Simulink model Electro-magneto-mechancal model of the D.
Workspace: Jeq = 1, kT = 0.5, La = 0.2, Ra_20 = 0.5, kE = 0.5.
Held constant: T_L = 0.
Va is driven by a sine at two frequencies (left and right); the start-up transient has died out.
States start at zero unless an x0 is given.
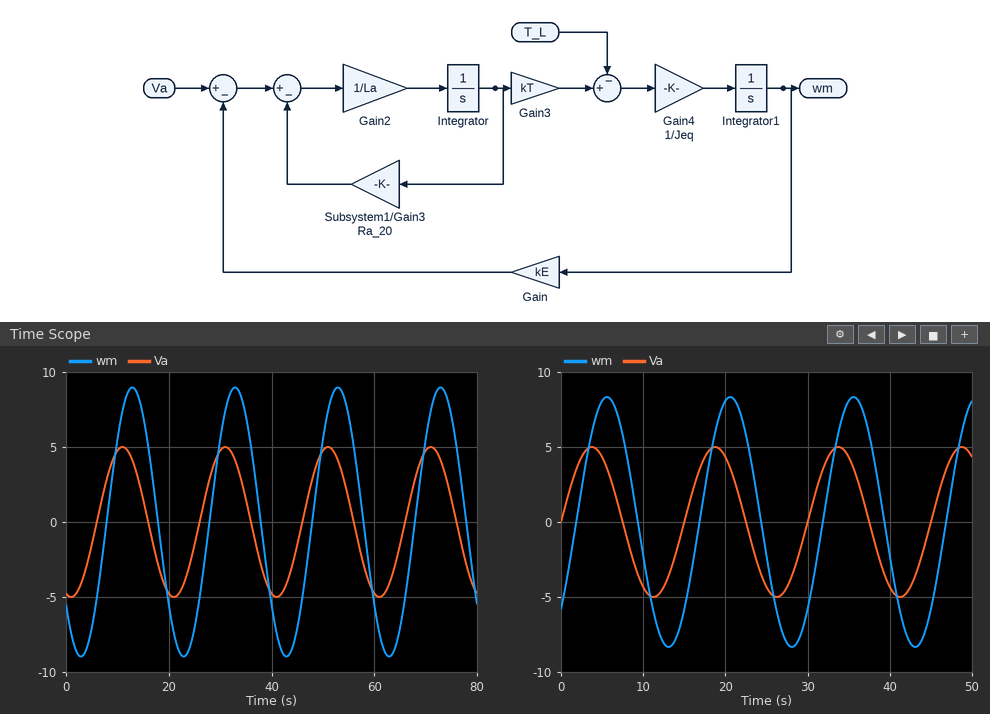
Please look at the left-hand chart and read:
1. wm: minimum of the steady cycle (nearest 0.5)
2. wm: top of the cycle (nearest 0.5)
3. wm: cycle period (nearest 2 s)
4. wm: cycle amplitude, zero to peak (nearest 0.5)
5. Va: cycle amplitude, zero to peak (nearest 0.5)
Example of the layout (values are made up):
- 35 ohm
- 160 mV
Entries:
- -9.0
- 9.0
- 20 s
- 9.0
- 5.0
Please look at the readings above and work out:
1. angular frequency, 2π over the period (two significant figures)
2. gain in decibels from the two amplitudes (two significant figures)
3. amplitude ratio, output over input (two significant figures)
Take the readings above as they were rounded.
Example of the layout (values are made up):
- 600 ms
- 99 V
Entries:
- 0.31 rad/s
- 5.1 dB
- 1.8
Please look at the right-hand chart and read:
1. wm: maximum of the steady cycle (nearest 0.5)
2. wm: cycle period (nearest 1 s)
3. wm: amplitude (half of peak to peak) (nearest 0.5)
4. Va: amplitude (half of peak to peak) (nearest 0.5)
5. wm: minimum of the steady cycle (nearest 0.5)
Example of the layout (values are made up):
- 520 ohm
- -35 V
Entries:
- 8.5
- 15 s
- 8.5
- 5.0
- -8.5
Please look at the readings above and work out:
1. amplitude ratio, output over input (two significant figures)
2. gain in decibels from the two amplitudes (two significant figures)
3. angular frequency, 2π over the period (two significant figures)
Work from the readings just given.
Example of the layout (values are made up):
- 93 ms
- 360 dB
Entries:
- 1.7
- 4.6 dB
- 0.42 rad/s
